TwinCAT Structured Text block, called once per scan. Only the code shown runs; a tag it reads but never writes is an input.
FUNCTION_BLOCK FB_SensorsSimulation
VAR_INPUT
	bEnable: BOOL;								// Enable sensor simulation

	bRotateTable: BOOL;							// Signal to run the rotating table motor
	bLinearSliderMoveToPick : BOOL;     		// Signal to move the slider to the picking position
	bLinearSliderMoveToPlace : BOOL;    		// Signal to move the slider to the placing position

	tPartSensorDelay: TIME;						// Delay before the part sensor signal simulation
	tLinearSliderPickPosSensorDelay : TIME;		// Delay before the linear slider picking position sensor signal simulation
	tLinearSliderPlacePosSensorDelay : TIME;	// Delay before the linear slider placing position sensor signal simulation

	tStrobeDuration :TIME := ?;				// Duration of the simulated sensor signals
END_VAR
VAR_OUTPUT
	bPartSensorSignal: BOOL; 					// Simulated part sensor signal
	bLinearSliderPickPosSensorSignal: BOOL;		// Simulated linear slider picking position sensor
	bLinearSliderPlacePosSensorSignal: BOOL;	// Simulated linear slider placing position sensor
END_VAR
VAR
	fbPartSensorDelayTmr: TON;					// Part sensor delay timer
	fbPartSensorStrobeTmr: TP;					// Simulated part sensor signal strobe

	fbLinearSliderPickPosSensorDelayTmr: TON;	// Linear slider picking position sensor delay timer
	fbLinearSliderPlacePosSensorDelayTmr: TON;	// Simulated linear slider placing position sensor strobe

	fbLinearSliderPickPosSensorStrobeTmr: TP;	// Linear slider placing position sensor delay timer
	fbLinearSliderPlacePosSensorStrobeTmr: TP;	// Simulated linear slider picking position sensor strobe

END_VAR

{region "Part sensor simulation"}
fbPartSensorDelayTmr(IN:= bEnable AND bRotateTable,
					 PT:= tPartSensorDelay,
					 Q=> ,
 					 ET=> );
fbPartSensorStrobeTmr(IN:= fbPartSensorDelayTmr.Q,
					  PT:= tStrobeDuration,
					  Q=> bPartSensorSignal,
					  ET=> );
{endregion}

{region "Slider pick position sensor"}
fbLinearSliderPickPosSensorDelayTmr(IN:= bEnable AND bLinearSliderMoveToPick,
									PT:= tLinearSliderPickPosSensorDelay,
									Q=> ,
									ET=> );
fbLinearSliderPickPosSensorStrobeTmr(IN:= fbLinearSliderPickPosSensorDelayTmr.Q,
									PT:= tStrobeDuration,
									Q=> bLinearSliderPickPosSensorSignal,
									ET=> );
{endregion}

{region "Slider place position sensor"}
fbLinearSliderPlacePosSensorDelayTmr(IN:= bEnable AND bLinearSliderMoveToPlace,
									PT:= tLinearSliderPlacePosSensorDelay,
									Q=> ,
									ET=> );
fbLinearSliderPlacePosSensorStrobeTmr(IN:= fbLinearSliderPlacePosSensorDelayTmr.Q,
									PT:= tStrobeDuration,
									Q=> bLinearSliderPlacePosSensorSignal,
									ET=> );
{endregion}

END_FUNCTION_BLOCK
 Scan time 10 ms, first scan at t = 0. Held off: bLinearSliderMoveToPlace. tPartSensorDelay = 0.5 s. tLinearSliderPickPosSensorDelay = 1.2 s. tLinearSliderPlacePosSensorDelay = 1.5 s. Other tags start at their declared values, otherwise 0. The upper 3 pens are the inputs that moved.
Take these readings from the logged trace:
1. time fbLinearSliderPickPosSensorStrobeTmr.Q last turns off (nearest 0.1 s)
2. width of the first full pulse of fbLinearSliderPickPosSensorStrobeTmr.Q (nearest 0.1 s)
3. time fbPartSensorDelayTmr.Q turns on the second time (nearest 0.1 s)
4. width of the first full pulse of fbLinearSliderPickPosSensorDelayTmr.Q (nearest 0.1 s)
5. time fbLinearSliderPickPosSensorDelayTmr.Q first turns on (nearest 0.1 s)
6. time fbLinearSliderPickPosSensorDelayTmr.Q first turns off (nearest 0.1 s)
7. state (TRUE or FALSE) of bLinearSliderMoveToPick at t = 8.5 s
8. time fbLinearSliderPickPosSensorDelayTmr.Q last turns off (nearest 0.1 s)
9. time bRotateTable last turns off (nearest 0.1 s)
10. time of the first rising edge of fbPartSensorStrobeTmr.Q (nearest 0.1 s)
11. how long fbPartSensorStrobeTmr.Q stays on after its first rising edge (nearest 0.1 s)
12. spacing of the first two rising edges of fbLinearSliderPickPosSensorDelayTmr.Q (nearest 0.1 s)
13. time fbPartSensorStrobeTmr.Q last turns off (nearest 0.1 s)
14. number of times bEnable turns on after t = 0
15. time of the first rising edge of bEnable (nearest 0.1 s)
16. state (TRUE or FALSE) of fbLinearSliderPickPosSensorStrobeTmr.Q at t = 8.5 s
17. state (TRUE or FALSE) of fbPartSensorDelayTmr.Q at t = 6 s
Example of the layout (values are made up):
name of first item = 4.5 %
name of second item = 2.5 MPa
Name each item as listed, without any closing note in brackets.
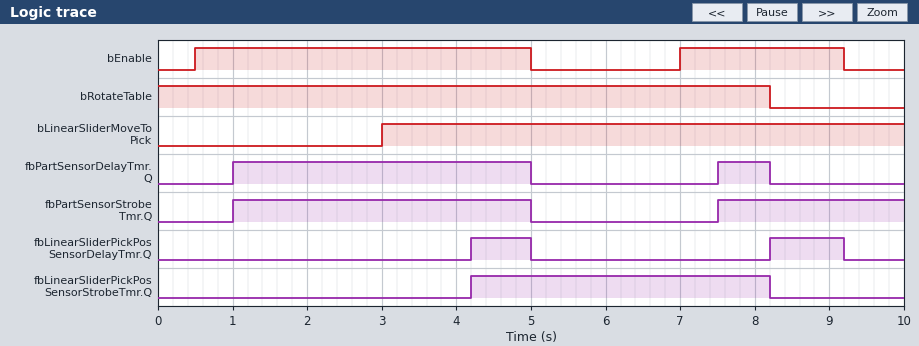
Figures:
time fbLinearSliderPickPosSensorStrobeTmr.Q last turns off = 8.2 s
width of the first full pulse of fbLinearSliderPickPosSensorStrobeTmr.Q = 4.0 s
time fbPartSensorDelayTmr.Q turns on the second time = 7.5 s
width of the first full pulse of fbLinearSliderPickPosSensorDelayTmr.Q = 0.8 s
time fbLinearSliderPickPosSensorDelayTmr.Q first turns on = 4.2 s
time fbLinearSliderPickPosSensorDelayTmr.Q first turns off = 5.0 s
state (TRUE or FALSE) of bLinearSliderMoveToPick at t = 8.5 s = TRUE
time fbLinearSliderPickPosSensorDelayTmr.Q last turns off = 9.2 s
time bRotateTable last turns off = 8.2 s
time of the first rising edge of fbPartSensorStrobeTmr.Q = 1.0 s
how long fbPartSensorStrobeTmr.Q stays on after its first rising edge = 4.0 s
spacing of the first two rising edges of fbLinearSliderPickPosSensorDelayTmr.Q = 4.0 s
time fbPartSensorStrobeTmr.Q last turns off = 5.0 s
number of times bEnable turns on after t = 0 = 2
time of the first rising edge of bEnable = 0.5 s
state (TRUE or FALSE) of fbLinearSliderPickPosSensorStrobeTmr.Q at t = 8.5 s = FALSE
state (TRUE or FALSE) of fbPartSensorDelayTmr.Q at t = 6 s = FALSE
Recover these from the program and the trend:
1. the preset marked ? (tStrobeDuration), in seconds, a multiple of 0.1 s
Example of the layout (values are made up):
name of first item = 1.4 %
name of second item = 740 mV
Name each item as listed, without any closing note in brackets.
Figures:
the preset marked ? (tStrobeDuration), in seconds, a multiple of 0.1 s = 4.0 s
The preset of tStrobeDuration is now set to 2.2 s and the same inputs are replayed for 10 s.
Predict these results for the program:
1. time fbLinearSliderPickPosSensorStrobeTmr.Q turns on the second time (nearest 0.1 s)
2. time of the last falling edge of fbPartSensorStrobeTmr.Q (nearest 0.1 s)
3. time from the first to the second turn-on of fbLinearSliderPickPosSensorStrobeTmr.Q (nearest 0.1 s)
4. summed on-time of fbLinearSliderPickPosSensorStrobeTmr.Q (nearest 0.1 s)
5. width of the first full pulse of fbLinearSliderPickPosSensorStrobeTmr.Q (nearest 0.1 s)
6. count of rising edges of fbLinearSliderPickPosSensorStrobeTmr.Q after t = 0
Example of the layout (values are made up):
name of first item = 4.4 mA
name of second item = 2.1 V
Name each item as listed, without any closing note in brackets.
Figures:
time fbLinearSliderPickPosSensorStrobeTmr.Q turns on the second time = 8.2 s
time of the last falling edge of fbPartSensorStrobeTmr.Q = 9.7 s
time from the first to the second turn-on of fbLinearSliderPickPosSensorStrobeTmr.Q = 4.0 s
summed on-time of fbLinearSliderPickPosSensorStrobeTmr.Q = 4.0 s
width of the first full pulse of fbLinearSliderPickPosSensorStrobeTmr.Q = 2.2 s
count of rising edges of fbLinearSliderPickPosSensorStrobeTmr.Q after t = 0 = 2
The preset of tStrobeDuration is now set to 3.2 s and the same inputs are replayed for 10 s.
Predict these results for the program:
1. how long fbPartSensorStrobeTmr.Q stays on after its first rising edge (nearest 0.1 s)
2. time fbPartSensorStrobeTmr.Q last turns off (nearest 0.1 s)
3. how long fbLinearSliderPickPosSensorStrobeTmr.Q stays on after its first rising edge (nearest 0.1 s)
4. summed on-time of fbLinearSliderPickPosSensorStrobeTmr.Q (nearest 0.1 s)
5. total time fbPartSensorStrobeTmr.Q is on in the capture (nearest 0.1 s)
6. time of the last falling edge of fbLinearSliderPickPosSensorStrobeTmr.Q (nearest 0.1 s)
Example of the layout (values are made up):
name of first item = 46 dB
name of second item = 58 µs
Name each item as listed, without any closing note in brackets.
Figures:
how long fbPartSensorStrobeTmr.Q stays on after its first rising edge = 3.2 s
time fbPartSensorStrobeTmr.Q last turns off = 4.2 s
how long fbLinearSliderPickPosSensorStrobeTmr.Q stays on after its first rising edge = 3.2 s
summed on-time of fbLinearSliderPickPosSensorStrobeTmr.Q = 5.0 s
total time fbPartSensorStrobeTmr.Q is on in the capture = 5.7 s
time of the last falling edge of fbLinearSliderPickPosSensorStrobeTmr.Q = 7.4 s
